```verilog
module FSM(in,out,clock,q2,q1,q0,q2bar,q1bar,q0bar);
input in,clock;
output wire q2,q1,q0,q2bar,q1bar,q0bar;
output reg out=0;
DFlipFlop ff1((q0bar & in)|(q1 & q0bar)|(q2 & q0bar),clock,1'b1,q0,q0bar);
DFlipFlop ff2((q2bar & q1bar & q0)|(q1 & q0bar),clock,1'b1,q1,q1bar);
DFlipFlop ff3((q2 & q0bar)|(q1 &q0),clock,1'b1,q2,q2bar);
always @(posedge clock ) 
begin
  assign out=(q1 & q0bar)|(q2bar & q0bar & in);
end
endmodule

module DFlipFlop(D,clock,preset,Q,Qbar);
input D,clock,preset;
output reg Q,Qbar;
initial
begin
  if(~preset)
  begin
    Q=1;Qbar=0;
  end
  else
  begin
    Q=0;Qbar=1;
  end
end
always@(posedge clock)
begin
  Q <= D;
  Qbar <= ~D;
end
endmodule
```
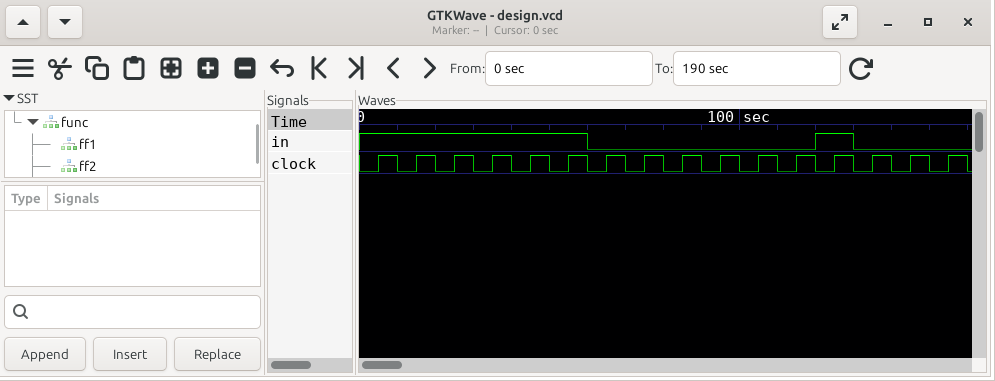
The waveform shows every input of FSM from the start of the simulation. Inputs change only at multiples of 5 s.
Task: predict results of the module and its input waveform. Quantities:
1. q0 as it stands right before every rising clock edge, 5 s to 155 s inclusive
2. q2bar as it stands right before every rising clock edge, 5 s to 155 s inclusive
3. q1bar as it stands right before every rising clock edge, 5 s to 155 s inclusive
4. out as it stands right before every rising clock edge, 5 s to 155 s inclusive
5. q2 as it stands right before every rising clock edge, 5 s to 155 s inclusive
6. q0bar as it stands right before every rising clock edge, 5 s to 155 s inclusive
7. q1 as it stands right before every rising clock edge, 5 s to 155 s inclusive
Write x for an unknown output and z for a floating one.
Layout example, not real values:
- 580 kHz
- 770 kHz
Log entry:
- 0 1 0 1 0 1 0 0 0 0 0 0 0 1 0 1
- 1 1 1 1 0 0 1 1 1 1 1 1 1 1 1 1
- 1 1 0 0 1 1 1 1 1 1 1 1 1 1 0 0
- 0 1 0 1 0 0 0 0 0 0 0 0 0 1 0 1
- 0 0 0 0 1 1 0 0 0 0 0 0 0 0 0 0
- 1 0 1 0 1 0 1 1 1 1 1 1 1 0 1 0
- 0 0 1 1 0 0 0 0 0 0 0 0 0 0 1 1
